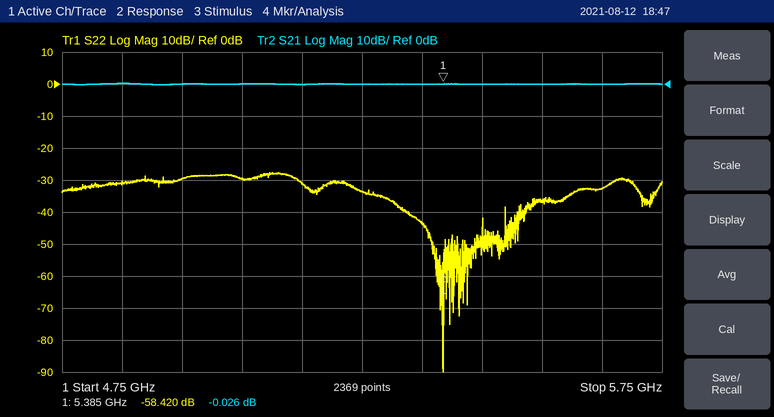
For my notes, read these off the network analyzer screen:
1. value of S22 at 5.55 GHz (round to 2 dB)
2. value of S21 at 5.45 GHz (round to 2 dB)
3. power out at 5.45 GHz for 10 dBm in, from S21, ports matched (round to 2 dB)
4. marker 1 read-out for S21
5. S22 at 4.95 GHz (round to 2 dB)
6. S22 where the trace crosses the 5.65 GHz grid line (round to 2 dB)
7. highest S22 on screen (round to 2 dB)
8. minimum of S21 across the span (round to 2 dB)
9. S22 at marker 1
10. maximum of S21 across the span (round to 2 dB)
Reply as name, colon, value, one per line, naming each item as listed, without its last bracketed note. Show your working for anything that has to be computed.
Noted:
value of S22 at 5.55 GHz: -36 dB
value of S21 at 5.45 GHz: 0 dB
power out at 5.45 GHz for 10 dBm in, from S21, ports matched: 10 dBm + (0 dB) = 10 dBm
marker 1 read-out for S21: -0.026 dB
S22 at 4.95 GHz: -30 dB
S22 where the trace crosses the 5.65 GHz grid line: -32 dB
highest S22 on screen: -28 dB
minimum of S21 across the span: 0 dB
S22 at marker 1: -58.420 dB
maximum of S21 across the span: 0 dB
